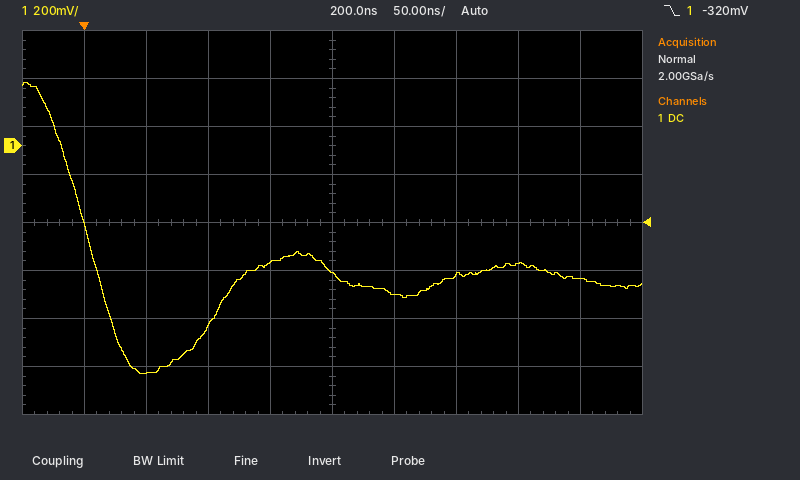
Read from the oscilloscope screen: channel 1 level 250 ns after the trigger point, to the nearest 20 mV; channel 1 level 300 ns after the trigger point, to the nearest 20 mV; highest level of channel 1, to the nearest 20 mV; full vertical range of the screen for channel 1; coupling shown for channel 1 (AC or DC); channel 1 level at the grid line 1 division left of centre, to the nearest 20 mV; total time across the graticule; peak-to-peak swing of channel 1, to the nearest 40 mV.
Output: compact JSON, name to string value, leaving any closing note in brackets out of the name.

{"channel 1 level 250 ns after the trigger point, to the nearest 20 mV": "-620 mV", "channel 1 level 300 ns after the trigger point, to the nearest 20 mV": "-540 mV", "highest level of channel 1, to the nearest 20 mV": "260 mV", "full vertical range of the screen for channel 1": "1.6 V", "coupling shown for channel 1": "DC", "channel 1 level at the grid line 1 division left of centre, to the nearest 20 mV": "-480 mV", "total time across the graticule": "500 ns", "peak-to-peak swing of channel 1, to the nearest 40 mV": "1.20 V"}
